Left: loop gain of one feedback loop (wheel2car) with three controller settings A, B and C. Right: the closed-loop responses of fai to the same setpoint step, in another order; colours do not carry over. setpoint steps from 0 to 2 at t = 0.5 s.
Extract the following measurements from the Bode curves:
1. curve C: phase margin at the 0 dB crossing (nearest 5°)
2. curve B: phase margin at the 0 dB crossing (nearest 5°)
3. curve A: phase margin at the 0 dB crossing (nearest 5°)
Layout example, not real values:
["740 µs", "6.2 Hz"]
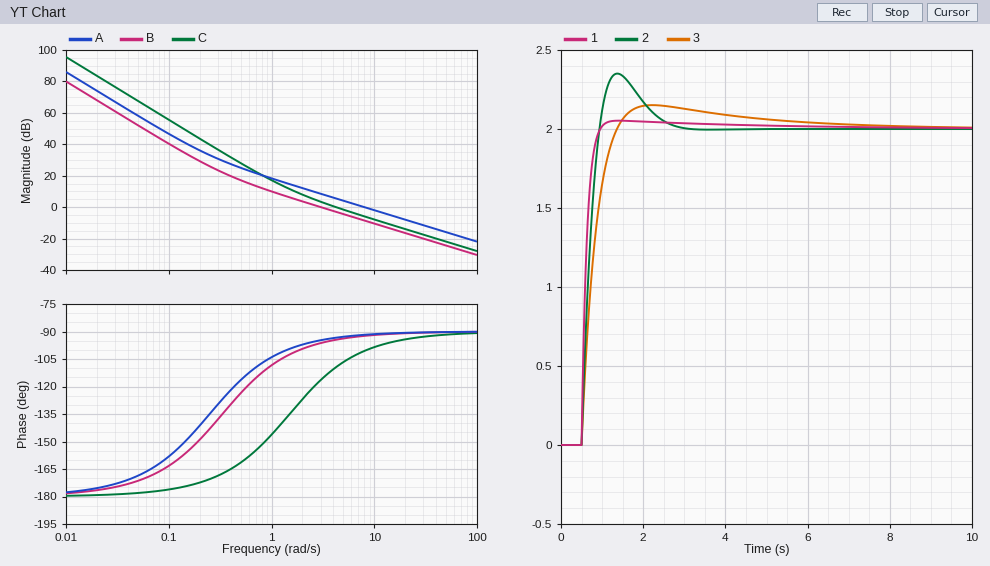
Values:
["70°", "85°", "90°"]
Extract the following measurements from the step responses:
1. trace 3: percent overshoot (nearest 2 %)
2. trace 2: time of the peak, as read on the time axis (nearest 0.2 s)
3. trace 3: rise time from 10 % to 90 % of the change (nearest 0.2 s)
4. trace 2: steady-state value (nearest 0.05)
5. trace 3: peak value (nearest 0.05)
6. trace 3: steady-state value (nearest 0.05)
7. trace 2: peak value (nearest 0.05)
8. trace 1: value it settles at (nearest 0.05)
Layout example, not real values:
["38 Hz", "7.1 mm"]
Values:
["8 %", "1.4 s", "0.6 s", "2.00", "2.15", "2.00", "2.35", "2.00"]
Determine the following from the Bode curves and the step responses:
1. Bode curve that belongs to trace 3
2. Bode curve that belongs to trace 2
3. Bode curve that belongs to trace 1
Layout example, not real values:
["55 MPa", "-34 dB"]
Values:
["B", "C", "A"]
